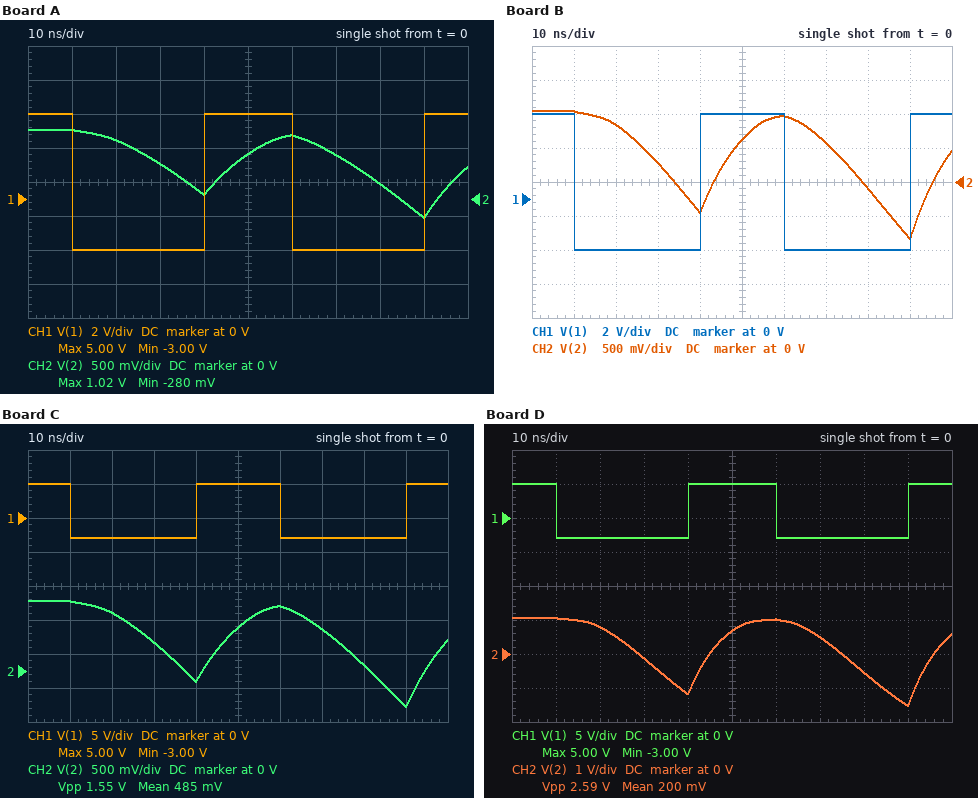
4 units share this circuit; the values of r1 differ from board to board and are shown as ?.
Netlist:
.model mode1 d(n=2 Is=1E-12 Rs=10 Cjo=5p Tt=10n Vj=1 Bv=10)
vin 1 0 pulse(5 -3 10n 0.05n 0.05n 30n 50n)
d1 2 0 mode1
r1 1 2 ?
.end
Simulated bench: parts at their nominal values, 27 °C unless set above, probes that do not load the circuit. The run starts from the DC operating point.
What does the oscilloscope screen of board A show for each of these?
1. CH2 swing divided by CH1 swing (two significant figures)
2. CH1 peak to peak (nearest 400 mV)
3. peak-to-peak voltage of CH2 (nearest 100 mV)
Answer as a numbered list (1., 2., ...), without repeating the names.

1. 0.16
2. 8.0 V
3. 1.3 V
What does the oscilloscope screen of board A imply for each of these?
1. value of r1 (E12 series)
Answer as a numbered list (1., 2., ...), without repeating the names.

1. 12 kΩ
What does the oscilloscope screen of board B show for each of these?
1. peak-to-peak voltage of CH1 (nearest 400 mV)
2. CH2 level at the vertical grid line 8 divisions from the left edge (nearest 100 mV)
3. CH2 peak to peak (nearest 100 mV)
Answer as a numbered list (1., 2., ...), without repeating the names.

1. 8.0 V
2. -100 mV
3. 1.9 V
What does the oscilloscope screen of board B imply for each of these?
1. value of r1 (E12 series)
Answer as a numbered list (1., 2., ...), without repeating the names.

1. 8.2 kΩ
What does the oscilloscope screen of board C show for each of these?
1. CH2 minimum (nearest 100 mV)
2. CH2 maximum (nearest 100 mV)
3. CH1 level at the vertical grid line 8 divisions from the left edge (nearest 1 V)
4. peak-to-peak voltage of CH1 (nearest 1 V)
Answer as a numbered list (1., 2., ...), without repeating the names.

1. -500 mV
2. 1.0 V
3. -3 V
4. 8 V
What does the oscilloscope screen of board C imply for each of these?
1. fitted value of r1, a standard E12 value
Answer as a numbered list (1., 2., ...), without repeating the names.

1. 10 kΩ
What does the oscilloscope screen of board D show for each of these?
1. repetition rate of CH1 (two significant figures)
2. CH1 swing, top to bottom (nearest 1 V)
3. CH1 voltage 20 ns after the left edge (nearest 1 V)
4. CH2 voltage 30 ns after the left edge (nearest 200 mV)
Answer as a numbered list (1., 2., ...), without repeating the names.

1. 20 MHz
2. 8 V
3. -3 V
4. -200 mV
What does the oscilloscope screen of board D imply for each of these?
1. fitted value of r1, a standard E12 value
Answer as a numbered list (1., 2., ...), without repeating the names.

1. 5.6 kΩ
